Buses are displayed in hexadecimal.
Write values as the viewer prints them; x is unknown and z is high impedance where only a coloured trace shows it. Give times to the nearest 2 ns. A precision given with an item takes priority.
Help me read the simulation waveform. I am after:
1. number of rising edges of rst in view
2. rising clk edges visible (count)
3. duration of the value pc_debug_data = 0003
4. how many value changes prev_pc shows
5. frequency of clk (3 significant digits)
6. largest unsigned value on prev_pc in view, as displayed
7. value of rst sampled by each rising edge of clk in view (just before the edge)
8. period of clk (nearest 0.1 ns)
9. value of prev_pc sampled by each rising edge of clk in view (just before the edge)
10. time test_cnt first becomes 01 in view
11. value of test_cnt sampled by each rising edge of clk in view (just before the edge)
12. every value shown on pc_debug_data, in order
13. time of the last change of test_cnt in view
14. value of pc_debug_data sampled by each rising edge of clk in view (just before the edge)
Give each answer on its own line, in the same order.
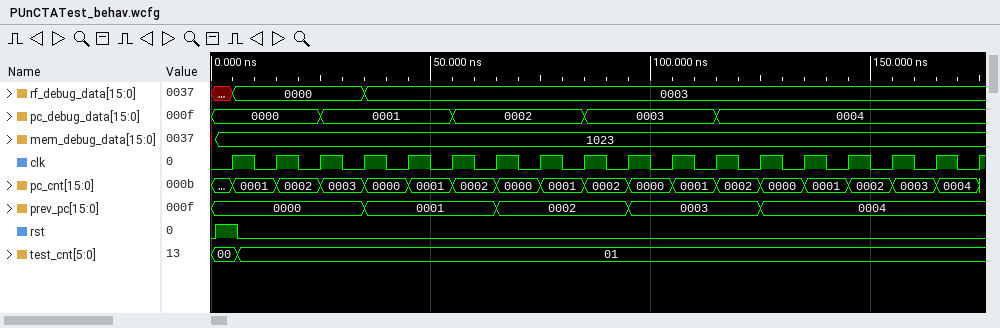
1
18
30 ns
4
100 MHz
0004
1 0 0 0 0 0 0 0 0 0 0 0 0 0 0 0 0 0
10 ns
0000, 0000, 0000, 0000, 0001, 0001, 0001, 0002, 0002, 0002, 0003, 0003, 0003, 0004, 0004, 0004, 0004, 0004
6 ns
00, 01, 01, 01, 01, 01, 01, 01, 01, 01, 01, 01, 01, 01, 01, 01, 01, 01
0000, 0001, 0002, 0003, 0004
6 ns
0000, 0000, 0000, 0001, 0001, 0001, 0002, 0002, 0002, 0003, 0003, 0003, 0004, 0004, 0004, 0004, 0004, 0004
